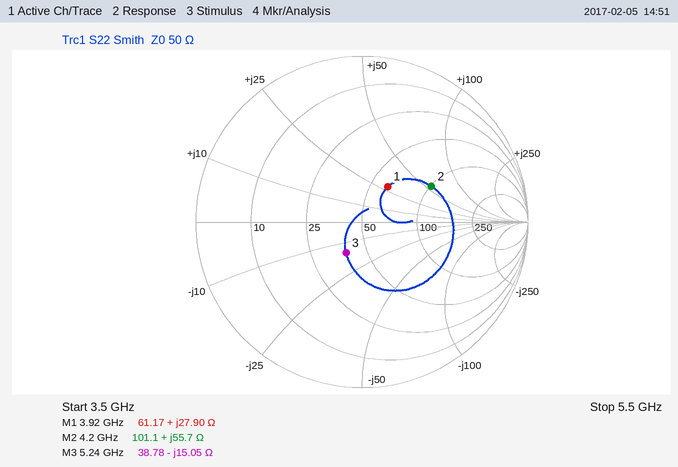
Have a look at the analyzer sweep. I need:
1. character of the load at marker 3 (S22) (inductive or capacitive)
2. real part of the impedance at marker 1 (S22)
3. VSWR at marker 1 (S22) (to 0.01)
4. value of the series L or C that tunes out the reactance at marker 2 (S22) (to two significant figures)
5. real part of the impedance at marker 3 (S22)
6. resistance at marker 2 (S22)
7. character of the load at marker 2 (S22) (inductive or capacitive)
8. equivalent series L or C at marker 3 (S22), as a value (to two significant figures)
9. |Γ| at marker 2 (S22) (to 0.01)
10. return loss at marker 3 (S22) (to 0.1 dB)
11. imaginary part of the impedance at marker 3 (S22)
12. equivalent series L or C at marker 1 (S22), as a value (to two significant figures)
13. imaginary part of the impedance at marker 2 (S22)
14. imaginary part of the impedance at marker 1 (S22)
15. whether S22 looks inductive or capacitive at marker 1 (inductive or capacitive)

capacitive
61.17 Ω
1.71
680 fF
38.78 Ω
101.1 Ω
inductive
2.0 pF
0.47
13.6 dB
-15.05 Ω
1.1 nH
+55.7 Ω
+27.90 Ω
inductive
